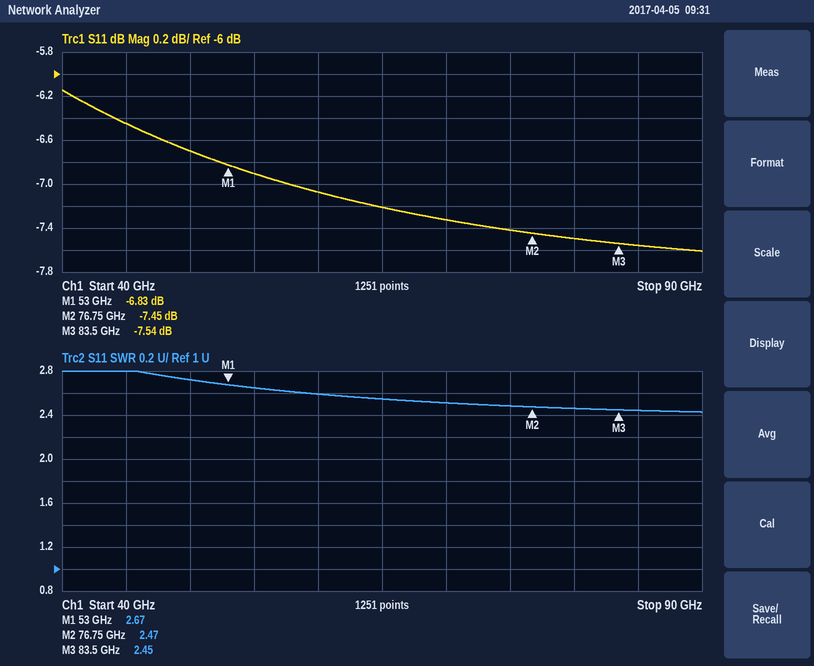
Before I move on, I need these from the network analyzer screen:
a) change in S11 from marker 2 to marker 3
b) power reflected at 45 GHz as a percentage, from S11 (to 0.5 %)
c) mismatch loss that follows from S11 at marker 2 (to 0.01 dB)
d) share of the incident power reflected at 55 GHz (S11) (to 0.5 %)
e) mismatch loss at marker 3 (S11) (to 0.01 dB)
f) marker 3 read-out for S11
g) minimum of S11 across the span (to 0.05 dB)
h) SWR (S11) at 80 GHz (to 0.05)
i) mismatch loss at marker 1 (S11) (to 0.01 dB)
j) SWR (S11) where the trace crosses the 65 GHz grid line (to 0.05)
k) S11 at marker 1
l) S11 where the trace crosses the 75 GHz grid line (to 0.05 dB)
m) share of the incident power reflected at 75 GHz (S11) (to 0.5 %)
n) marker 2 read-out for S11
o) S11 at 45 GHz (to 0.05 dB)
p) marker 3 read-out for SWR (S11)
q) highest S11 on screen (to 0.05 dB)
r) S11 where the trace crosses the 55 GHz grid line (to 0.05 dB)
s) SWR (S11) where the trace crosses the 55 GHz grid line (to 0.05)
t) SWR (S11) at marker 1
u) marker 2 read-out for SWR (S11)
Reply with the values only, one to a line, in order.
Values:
-0.09 dB
22.5 %
0.86 dB
20.5 %
0.84 dB
-7.54 dB
-7.60 dB
2.45
1.01 dB
2.55
-6.83 dB
-7.40 dB
18.0 %
-7.45 dB
-6.45 dB
2.45
-6.15 dB
-6.90 dB
2.65
2.67
2.47
